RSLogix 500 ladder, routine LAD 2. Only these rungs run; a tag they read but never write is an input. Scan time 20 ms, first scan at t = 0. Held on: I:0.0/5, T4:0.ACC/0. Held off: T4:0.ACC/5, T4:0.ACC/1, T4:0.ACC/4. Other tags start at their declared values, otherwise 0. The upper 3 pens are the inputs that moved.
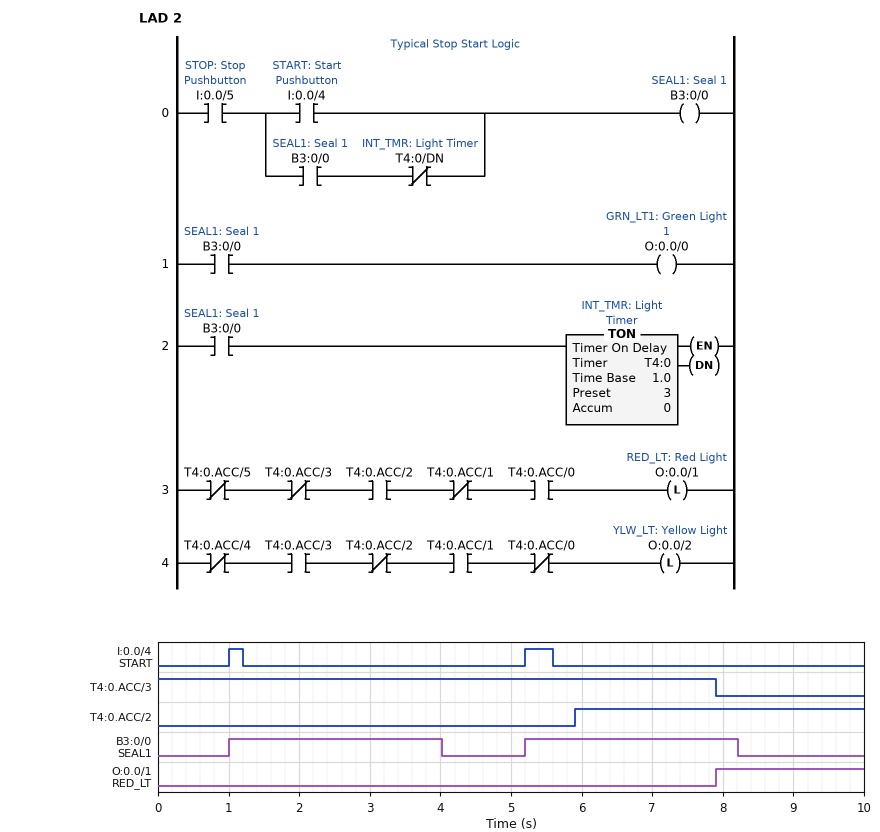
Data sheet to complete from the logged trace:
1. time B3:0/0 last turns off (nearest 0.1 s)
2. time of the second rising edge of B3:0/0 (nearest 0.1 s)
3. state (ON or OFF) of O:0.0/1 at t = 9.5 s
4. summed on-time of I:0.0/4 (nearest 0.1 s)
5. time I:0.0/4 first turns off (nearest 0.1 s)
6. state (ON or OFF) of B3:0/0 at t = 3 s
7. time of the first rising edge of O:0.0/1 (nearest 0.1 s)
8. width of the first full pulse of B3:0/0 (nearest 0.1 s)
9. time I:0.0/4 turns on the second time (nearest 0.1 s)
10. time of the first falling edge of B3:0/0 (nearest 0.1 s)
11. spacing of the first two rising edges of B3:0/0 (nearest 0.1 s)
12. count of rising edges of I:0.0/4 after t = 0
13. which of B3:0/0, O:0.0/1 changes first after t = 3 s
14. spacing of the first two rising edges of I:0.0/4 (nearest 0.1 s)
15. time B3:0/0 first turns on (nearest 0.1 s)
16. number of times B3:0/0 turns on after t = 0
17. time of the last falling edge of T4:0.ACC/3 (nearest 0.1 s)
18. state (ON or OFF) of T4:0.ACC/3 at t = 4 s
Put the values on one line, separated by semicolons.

8.2 s; 5.2 s; ON; 0.6 s; 1.2 s; ON; 7.9 s; 3.0 s; 5.2 s; 4.0 s; 4.2 s; 2; B3:0/0; 4.2 s; 1.0 s; 2; 7.9 s; ON
